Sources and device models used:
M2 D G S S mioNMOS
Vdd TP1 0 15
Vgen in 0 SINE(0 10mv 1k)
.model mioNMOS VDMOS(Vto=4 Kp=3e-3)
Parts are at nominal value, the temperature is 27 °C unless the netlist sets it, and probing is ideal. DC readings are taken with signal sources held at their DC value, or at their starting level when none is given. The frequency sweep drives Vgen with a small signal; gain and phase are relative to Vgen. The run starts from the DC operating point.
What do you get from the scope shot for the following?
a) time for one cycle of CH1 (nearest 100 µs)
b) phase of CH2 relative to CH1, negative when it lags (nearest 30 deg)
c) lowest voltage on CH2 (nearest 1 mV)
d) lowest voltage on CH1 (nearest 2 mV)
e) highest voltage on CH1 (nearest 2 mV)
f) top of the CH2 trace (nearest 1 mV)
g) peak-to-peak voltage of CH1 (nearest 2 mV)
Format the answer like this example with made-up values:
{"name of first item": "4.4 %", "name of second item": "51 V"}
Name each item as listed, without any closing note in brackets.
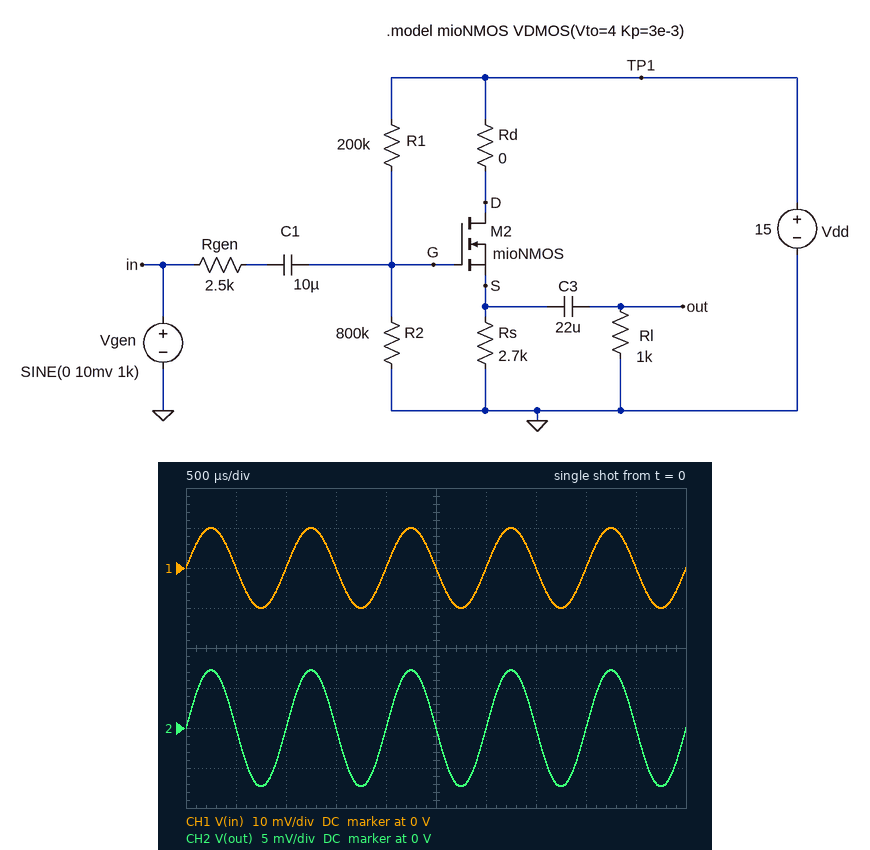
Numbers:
{"time for one cycle of CH1": "1.0 ms", "phase of CH2 relative to CH1, negative when it lags": "0 deg", "lowest voltage on CH2": "-7 mV", "lowest voltage on CH1": "-10 mV", "highest voltage on CH1": "10 mV", "top of the CH2 trace": "7 mV", "peak-to-peak voltage of CH1": "20 mV"}
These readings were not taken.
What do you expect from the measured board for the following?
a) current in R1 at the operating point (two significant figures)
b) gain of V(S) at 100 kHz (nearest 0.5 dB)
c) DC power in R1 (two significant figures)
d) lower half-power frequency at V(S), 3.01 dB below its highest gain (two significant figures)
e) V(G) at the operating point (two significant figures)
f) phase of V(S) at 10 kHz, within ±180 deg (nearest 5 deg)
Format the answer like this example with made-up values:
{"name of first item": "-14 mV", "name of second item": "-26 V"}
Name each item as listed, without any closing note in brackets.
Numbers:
{"current in R1 at the operating point": "15 µA", "gain of V(S) at 100 kHz": "-6.0 dB", "DC power in R1": "45 µW", "lower half-power frequency at V(S), 3.01 dB below its highest gain": "96 mHz", "V(G) at the operating point": "12 V", "phase of V(S) at 10 kHz, within ±180 deg": "-5 deg"}
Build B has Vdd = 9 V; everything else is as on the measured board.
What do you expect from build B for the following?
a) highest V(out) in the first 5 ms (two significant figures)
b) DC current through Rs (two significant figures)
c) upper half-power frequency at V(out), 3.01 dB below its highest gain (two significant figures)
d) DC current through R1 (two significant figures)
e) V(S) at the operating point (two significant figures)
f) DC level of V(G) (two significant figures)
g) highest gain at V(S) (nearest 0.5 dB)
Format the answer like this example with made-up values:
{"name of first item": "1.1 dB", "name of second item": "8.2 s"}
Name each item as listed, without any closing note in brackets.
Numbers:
{"highest V(out) in the first 5 ms": "6.2 mV", "DC current through Rs": "900 µA", "upper half-power frequency at V(out), 3.01 dB below its highest gain": "68 kHz", "DC current through R1": "9.0 µA", "V(S) at the operating point": "2.4 V", "DC level of V(G)": "7.2 V", "highest gain at V(S)": "-1.5 dB"}
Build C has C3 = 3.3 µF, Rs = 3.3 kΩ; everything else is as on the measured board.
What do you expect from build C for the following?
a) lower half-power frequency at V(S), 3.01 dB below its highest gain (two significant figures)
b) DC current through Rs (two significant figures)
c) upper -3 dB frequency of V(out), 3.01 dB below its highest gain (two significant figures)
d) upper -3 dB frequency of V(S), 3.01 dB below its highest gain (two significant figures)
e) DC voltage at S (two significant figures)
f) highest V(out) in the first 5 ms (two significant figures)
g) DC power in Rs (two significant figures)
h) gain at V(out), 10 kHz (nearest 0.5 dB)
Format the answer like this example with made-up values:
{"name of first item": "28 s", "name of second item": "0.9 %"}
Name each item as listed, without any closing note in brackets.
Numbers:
{"lower half-power frequency at V(S), 3.01 dB below its highest gain": "98 mHz", "DC current through Rs": "2.1 mA", "upper -3 dB frequency of V(out), 3.01 dB below its highest gain": "96 kHz", "upper -3 dB frequency of V(S), 3.01 dB below its highest gain": "48 kHz", "DC voltage at S": "6.8 V", "highest V(out) in the first 5 ms": "7.1 mV", "DC power in Rs": "14 mW", "gain at V(out), 10 kHz": "-3.0 dB"}
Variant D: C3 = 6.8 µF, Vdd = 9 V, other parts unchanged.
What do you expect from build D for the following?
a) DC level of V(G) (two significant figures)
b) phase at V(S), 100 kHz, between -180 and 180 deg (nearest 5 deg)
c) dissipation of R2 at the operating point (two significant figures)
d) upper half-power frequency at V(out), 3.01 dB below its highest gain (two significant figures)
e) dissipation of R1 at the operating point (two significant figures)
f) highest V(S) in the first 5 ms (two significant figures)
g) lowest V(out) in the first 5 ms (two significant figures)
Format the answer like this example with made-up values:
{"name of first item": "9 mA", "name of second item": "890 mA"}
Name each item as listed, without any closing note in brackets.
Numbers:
{"DC level of V(G)": "7.2 V", "phase at V(S), 100 kHz, between -180 and 180 deg": "-45 deg", "dissipation of R2 at the operating point": "65 µW", "upper half-power frequency at V(out), 3.01 dB below its highest gain": "68 kHz", "dissipation of R1 at the operating point": "16 µW", "highest V(S) in the first 5 ms": "2.4 V", "lowest V(out) in the first 5 ms": "-6.3 mV"}
